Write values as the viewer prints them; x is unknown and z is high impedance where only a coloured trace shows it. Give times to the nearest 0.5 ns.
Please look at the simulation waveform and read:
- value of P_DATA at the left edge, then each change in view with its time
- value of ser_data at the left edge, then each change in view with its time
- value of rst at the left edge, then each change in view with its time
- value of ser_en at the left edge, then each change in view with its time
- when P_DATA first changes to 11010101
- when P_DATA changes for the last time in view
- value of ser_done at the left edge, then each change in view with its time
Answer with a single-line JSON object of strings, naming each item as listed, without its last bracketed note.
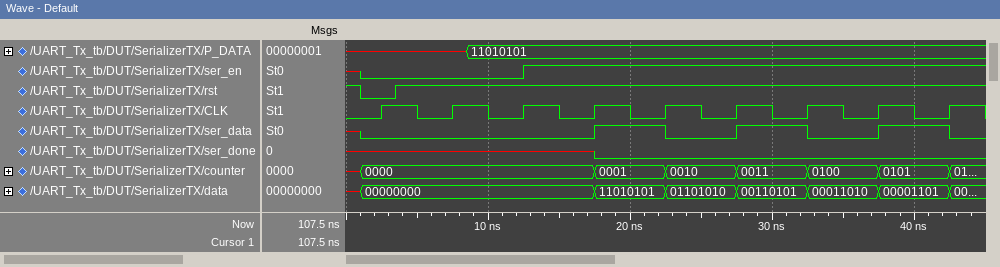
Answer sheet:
{"value of P_DATA at the left edge, then each change in view with its time": "x, 11010101 at 8.5 ns", "value of ser_data at the left edge, then each change in view with its time": "x, 0 at 1 ns, 1 at 17.5 ns, 0 at 22.5 ns, 1 at 27.5 ns, 0 at 32.5 ns, 1 at 37.5 ns, 0 at 42.5 ns", "value of rst at the left edge, then each change in view with its time": "1, 0 at 1 ns, 1 at 3.5 ns", "value of ser_en at the left edge, then each change in view with its time": "x, 0 at 1 ns, 1 at 12.5 ns", "when P_DATA first changes to 11010101": "8.5 ns", "when P_DATA changes for the last time in view": "8.5 ns", "value of ser_done at the left edge, then each change in view with its time": "x, 0 at 17.5 ns"}
